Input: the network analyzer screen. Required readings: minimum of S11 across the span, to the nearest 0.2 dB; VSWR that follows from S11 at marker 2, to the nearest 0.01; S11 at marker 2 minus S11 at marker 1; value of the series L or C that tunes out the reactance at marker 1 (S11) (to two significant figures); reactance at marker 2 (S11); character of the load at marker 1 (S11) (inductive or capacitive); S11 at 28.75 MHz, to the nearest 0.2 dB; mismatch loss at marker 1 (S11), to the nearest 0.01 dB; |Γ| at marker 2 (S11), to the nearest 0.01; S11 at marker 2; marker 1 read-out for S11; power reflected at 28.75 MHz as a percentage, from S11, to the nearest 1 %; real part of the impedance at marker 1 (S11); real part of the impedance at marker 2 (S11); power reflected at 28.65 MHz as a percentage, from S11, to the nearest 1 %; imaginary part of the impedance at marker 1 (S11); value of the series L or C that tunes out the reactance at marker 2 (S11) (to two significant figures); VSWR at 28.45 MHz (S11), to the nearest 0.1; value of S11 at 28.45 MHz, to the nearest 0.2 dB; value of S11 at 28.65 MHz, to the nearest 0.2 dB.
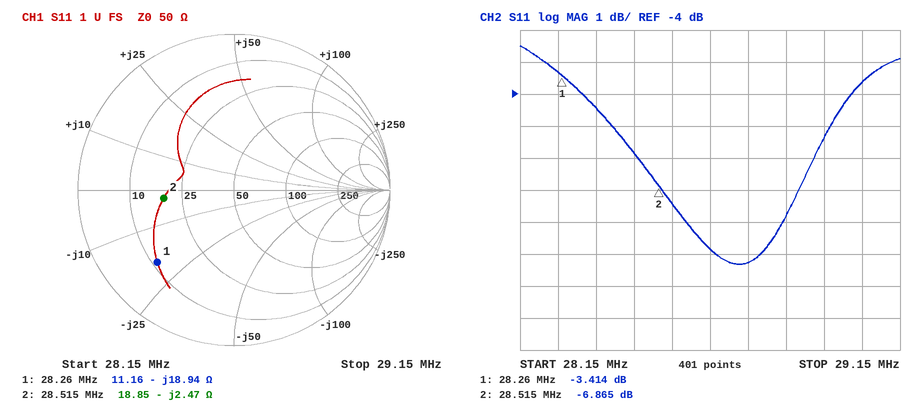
-9.4 dB
2.66
-3.451 dB
110 nH
-2.47 Ω
capacitive
-9.2 dB
2.64 dB
0.45
-6.865 dB
-3.414 dB
12 %
11.16 Ω
18.85 Ω
13 %
-18.94 Ω
14 nH
3.1
-5.8 dB
-8.8 dB
